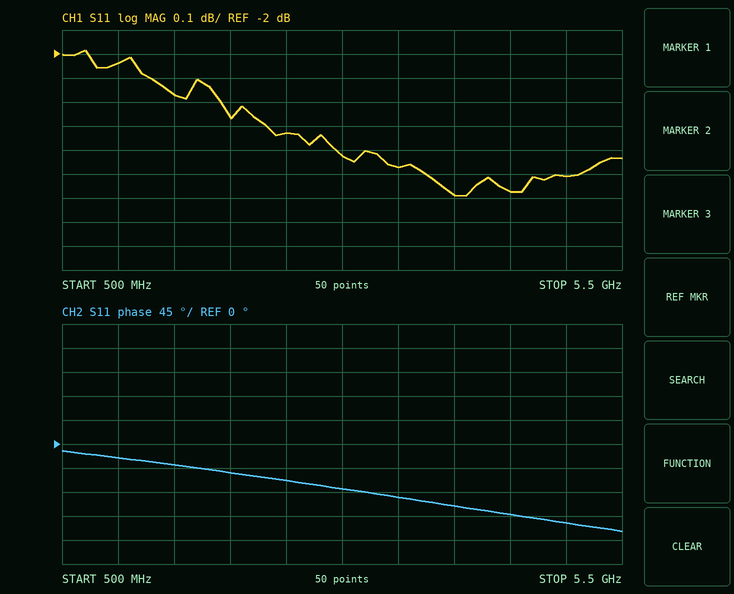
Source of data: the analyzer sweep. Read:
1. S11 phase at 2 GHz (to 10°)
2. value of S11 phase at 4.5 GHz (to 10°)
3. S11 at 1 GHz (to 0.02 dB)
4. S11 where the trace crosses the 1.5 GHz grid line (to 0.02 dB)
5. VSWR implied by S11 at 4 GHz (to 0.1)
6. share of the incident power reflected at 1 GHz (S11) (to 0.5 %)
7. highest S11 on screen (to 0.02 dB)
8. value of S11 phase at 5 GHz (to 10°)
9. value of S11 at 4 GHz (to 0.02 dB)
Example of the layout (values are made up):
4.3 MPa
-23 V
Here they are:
-50°
-130°
-2.04 dB
-2.16 dB
6.8
62.5 %
-1.98 dB
-150°
-2.58 dB
